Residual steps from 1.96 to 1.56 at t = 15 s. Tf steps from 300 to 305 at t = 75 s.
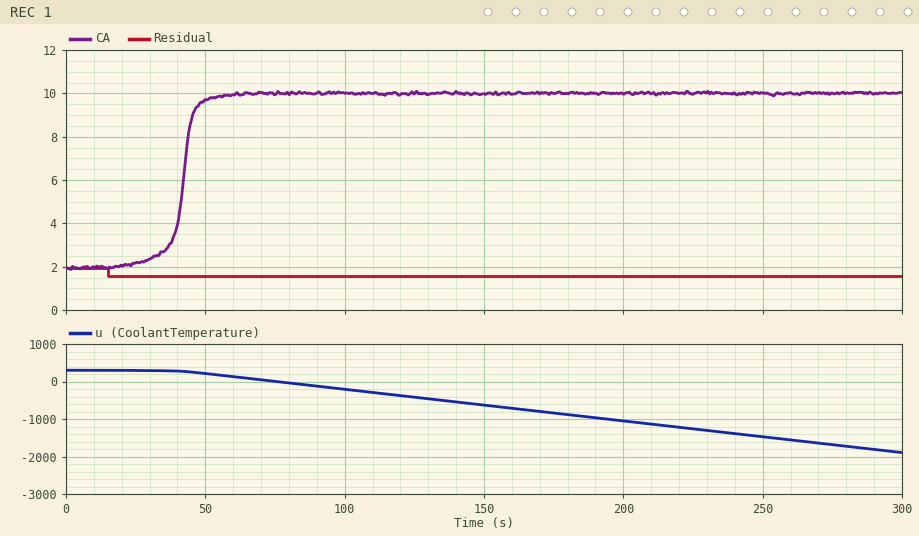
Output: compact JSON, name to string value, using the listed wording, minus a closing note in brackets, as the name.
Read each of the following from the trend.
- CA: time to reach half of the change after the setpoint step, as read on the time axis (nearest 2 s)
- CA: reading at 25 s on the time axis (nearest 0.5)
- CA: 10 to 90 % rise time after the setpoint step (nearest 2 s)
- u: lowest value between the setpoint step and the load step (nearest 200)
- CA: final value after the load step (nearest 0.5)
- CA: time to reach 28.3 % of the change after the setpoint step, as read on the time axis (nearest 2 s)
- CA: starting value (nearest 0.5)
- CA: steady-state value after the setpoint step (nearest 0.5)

{"CA: time to reach half of the change after the setpoint step, as read on the time axis": "42 s", "CA: reading at 25 s on the time axis": "2.0", "CA: 10 to 90 % rise time after the setpoint step": "10 s", "u: lowest value between the setpoint step and the load step": "0", "CA: final value after the load step": "10.0", "CA: time to reach 28.3 % of the change after the setpoint step, as read on the time axis": "40 s", "CA: starting value": "2.0", "CA: steady-state value after the setpoint step": "10.0"}
